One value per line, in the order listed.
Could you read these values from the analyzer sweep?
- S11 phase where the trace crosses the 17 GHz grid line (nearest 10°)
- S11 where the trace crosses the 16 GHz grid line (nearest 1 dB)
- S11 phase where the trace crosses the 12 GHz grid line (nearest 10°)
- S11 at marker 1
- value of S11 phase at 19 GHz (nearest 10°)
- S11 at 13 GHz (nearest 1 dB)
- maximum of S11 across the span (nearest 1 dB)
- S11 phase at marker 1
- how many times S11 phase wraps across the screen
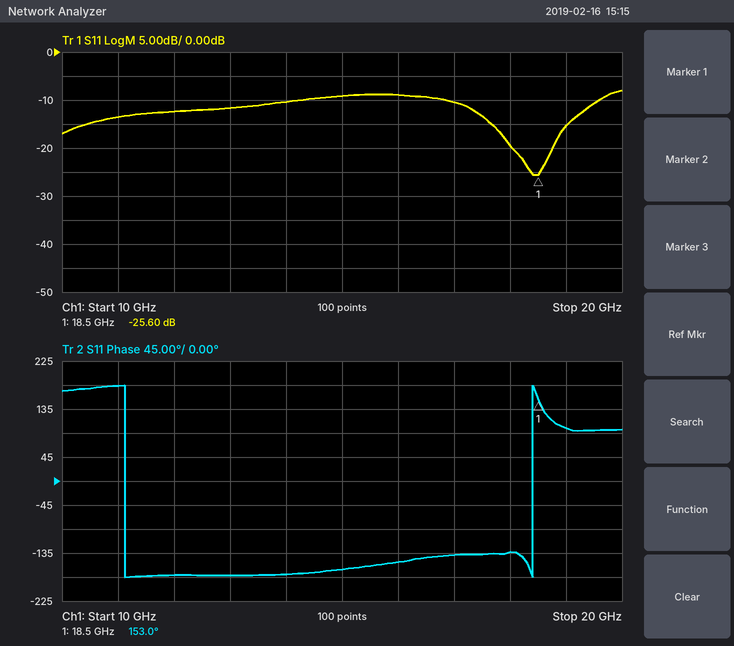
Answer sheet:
-140°
-9 dB
-180°
-25.60 dB
100°
-12 dB
-8 dB
153.0°
2
